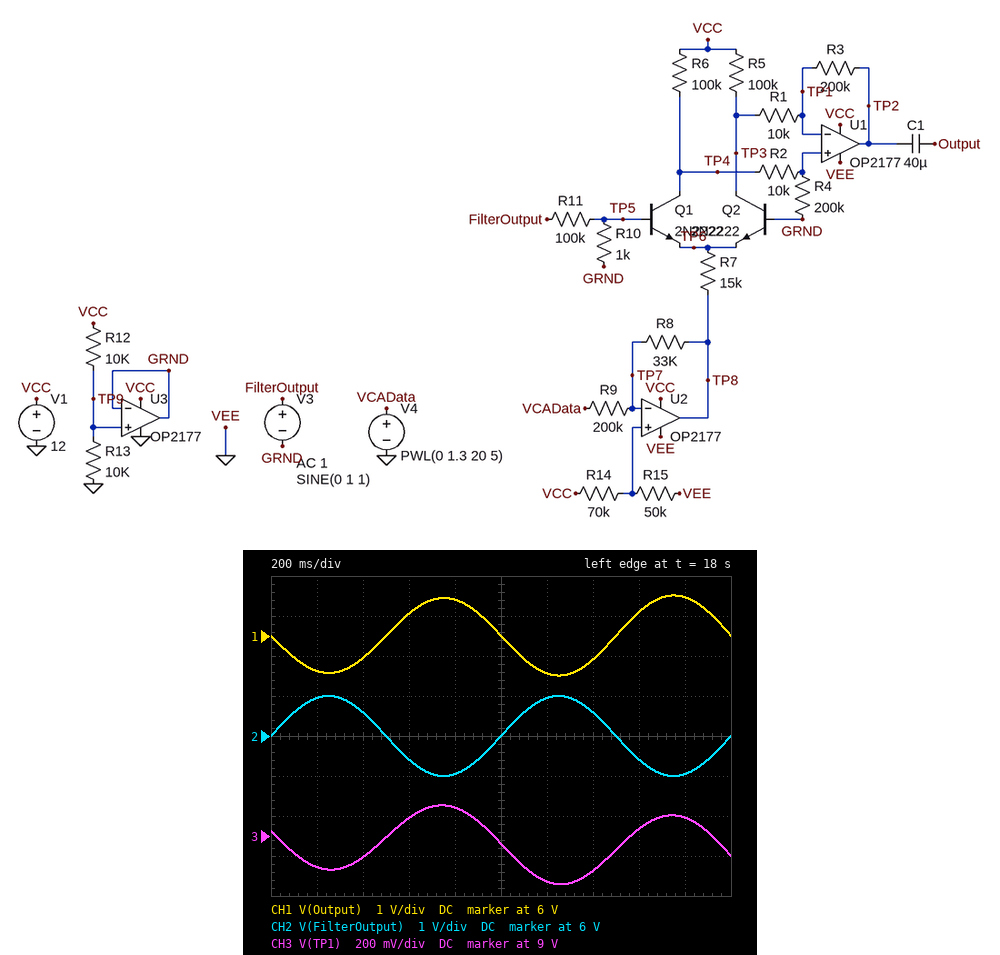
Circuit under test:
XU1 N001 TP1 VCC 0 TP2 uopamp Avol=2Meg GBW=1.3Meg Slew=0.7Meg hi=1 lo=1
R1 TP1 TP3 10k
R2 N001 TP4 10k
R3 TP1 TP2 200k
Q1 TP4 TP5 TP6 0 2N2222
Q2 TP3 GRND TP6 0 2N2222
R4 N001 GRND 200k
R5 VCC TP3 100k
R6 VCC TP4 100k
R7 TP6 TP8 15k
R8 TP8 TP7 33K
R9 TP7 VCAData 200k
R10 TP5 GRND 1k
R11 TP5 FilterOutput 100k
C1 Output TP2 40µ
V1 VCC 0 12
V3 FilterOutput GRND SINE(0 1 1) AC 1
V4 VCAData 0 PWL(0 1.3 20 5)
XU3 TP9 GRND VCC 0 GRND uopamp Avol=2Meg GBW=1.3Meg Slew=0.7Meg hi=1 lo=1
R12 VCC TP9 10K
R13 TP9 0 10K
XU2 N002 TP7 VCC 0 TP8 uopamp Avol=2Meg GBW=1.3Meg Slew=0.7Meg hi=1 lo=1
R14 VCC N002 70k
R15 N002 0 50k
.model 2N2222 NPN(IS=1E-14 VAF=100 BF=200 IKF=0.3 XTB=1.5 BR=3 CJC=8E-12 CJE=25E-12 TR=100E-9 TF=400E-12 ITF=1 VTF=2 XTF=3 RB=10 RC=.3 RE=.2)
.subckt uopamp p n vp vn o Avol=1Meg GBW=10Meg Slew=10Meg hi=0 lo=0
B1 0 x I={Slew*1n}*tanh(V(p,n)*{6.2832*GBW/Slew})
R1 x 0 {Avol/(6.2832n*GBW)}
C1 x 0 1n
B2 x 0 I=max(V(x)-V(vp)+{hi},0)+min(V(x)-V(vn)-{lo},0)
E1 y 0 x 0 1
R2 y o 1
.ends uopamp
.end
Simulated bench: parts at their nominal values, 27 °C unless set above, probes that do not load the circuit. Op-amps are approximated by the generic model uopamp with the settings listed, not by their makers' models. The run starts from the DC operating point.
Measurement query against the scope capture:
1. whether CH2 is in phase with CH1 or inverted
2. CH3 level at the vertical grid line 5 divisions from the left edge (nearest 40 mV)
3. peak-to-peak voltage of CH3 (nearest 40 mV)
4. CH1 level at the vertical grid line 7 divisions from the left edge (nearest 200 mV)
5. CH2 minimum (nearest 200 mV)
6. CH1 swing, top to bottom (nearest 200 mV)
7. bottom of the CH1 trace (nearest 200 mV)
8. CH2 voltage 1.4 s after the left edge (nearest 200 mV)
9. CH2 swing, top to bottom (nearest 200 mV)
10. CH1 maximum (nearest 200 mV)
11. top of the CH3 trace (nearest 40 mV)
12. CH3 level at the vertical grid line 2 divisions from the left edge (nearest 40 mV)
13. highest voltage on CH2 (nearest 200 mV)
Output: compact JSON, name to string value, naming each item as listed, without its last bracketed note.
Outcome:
{"whether CH2 is in phase with CH1 or inverted": "inverted", "CH3 level at the vertical grid line 5 divisions from the left edge": "8.96 V", "peak-to-peak voltage of CH3": "400 mV", "CH1 level at the vertical grid line 7 divisions from the left edge": "5.4 V", "CH2 minimum": "5.0 V", "CH1 swing, top to bottom": "2.0 V", "bottom of the CH1 trace": "5.0 V", "CH2 voltage 1.4 s after the left edge": "6.6 V", "CH2 swing, top to bottom": "2.0 V", "CH1 maximum": "7.0 V", "top of the CH3 trace": "9.16 V", "CH3 level at the vertical grid line 2 divisions from the left edge": "8.88 V", "highest voltage on CH2": "7.0 V"}
